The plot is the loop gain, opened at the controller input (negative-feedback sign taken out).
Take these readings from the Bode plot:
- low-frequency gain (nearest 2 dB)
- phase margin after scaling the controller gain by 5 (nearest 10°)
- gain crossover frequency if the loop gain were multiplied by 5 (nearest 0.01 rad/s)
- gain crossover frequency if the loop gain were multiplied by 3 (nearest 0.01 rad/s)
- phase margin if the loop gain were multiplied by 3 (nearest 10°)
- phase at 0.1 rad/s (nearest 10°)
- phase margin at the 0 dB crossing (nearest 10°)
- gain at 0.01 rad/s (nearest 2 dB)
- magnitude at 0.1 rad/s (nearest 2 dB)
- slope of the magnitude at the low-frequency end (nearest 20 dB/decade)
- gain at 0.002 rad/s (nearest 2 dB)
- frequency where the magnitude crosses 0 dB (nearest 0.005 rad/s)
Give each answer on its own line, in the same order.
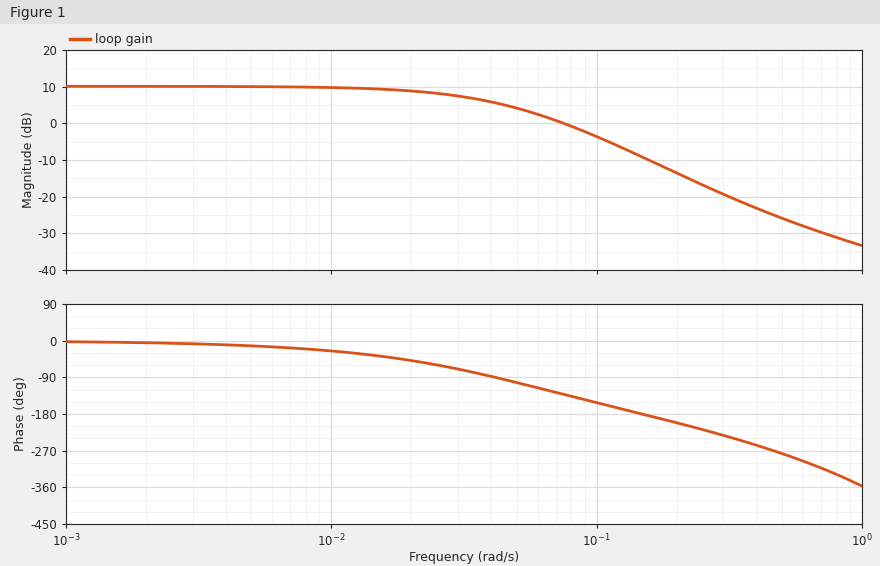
10 dB
-20°
0.21 rad/s
0.15 rad/s
0°
-150°
50°
10 dB
-4 dB
0 dB/decade
10 dB
0.075 rad/s
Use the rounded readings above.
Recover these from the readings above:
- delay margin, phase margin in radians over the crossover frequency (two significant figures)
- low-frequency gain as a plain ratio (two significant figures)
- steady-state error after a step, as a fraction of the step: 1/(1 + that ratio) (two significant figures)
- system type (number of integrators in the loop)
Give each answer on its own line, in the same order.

12 s
3.2
0.24
0
